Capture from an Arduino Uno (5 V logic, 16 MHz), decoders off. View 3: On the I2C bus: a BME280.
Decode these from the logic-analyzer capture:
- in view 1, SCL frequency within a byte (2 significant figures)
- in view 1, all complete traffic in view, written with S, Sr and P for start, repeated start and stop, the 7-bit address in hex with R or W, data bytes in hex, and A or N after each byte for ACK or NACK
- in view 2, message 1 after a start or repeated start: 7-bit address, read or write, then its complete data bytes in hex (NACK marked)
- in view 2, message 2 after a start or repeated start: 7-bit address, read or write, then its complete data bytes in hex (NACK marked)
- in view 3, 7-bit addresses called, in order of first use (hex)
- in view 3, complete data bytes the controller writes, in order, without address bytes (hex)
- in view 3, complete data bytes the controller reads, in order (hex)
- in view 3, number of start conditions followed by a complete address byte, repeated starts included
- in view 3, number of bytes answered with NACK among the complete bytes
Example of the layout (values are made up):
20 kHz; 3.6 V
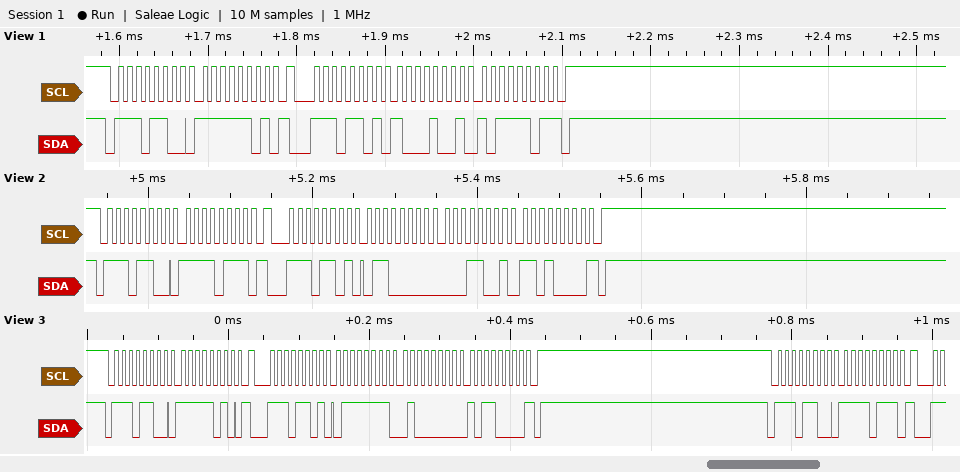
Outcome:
100 kHz; S 76W A FD A Sr 76R A 89 A BD N P; 0x76 write: F7; 0x76 read: 60 19 D0 NACK; 0x76; FA F7; 7F 40 B0; 3; 1
